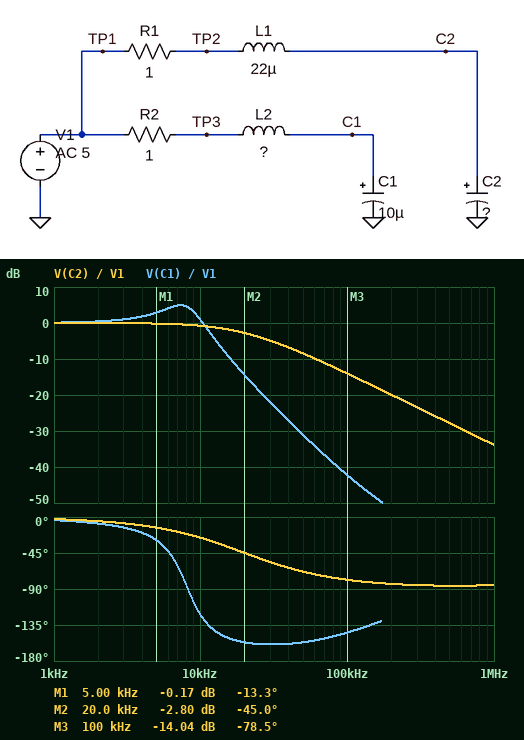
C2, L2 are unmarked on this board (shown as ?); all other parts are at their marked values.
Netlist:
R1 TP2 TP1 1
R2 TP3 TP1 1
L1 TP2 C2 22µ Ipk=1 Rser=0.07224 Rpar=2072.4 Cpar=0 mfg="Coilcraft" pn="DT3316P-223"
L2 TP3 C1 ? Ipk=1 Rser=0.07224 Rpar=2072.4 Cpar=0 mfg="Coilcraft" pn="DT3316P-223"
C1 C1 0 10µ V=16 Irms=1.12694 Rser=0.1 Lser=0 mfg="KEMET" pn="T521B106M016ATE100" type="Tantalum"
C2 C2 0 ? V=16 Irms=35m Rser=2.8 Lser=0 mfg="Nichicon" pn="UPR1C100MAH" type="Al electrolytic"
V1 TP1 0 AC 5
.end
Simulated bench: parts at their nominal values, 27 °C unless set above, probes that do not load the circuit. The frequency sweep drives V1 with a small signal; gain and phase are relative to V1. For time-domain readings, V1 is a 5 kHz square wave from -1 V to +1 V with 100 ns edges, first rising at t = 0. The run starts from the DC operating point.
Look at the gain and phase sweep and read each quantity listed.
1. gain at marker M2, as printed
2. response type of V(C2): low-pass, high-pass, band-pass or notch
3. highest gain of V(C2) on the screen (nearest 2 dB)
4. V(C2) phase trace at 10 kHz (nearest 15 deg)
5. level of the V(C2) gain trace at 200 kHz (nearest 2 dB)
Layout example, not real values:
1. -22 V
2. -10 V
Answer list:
1. -2.80 dB
2. low-pass
3. 0 dB
4. -30 deg
5. -20 dB
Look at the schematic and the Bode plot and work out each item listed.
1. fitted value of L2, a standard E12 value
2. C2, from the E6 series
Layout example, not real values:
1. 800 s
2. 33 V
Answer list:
1. 39 µH
2. 6.8 µF
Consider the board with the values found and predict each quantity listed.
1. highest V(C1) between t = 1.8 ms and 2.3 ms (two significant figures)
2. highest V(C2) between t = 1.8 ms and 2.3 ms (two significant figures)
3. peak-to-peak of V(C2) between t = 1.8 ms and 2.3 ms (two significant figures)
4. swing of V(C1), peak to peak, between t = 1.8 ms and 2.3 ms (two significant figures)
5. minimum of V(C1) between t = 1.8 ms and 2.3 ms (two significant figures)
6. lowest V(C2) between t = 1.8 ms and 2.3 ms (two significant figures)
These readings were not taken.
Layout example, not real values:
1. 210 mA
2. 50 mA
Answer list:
1. 1.8 V
2. 1.0 V
3. 2.0 V
4. 3.5 V
5. -1.8 V
6. -1.0 V
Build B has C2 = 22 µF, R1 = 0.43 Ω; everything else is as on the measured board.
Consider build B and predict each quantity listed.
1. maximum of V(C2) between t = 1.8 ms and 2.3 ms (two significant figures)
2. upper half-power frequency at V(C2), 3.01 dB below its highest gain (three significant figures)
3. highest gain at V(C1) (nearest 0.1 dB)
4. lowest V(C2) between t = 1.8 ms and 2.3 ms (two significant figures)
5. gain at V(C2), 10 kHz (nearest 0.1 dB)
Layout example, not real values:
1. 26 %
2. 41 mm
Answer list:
1. 980 mV
2. 19.0 kHz
3. 4.9 dB
4. -980 mV
5. -1.3 dB
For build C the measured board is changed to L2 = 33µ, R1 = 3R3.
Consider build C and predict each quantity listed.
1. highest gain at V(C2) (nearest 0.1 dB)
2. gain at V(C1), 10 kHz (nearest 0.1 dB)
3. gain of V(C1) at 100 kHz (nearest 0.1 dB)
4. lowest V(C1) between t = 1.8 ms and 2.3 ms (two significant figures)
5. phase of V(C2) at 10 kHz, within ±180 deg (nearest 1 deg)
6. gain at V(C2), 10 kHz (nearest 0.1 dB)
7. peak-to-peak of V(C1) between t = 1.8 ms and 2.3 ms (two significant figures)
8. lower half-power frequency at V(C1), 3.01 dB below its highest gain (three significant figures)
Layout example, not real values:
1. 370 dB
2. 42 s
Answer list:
1. 0 dB
2. 2.0 dB
3. -40.8 dB
4. -1.7 V
5. -31 deg
6. -4.7 dB
7. 3.3 V
8. 3.73 kHz
